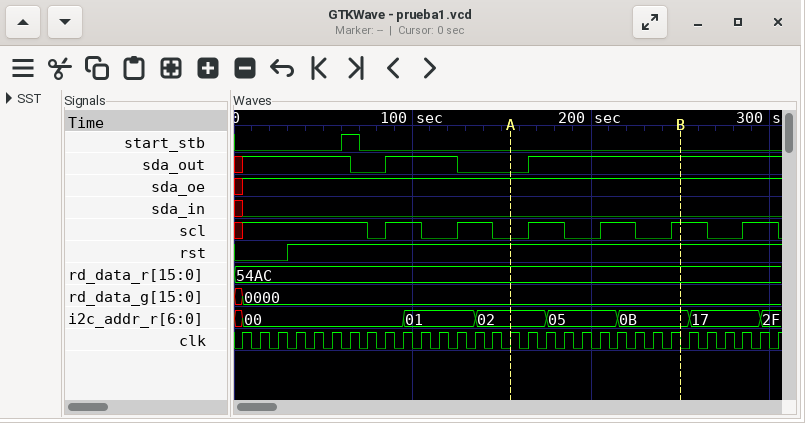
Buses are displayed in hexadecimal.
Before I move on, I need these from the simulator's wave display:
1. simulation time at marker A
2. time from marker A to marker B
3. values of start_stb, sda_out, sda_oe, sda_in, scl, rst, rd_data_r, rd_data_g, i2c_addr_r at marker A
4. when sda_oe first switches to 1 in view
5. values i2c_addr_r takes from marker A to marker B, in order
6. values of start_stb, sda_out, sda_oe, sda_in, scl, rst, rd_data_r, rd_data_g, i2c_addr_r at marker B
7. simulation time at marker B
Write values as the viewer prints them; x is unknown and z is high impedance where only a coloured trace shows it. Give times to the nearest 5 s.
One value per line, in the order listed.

155 s
95 s
start_stb=0, sda_out=0, sda_oe=1, sda_in=0, scl=0, rst=1, rd_data_r=54AC, rd_data_g=0000, i2c_addr_r=02
5 s
02, 05, 0B
start_stb=0, sda_out=1, sda_oe=1, sda_in=0, scl=1, rst=1, rd_data_r=54AC, rd_data_g=0000, i2c_addr_r=0B
250 s
